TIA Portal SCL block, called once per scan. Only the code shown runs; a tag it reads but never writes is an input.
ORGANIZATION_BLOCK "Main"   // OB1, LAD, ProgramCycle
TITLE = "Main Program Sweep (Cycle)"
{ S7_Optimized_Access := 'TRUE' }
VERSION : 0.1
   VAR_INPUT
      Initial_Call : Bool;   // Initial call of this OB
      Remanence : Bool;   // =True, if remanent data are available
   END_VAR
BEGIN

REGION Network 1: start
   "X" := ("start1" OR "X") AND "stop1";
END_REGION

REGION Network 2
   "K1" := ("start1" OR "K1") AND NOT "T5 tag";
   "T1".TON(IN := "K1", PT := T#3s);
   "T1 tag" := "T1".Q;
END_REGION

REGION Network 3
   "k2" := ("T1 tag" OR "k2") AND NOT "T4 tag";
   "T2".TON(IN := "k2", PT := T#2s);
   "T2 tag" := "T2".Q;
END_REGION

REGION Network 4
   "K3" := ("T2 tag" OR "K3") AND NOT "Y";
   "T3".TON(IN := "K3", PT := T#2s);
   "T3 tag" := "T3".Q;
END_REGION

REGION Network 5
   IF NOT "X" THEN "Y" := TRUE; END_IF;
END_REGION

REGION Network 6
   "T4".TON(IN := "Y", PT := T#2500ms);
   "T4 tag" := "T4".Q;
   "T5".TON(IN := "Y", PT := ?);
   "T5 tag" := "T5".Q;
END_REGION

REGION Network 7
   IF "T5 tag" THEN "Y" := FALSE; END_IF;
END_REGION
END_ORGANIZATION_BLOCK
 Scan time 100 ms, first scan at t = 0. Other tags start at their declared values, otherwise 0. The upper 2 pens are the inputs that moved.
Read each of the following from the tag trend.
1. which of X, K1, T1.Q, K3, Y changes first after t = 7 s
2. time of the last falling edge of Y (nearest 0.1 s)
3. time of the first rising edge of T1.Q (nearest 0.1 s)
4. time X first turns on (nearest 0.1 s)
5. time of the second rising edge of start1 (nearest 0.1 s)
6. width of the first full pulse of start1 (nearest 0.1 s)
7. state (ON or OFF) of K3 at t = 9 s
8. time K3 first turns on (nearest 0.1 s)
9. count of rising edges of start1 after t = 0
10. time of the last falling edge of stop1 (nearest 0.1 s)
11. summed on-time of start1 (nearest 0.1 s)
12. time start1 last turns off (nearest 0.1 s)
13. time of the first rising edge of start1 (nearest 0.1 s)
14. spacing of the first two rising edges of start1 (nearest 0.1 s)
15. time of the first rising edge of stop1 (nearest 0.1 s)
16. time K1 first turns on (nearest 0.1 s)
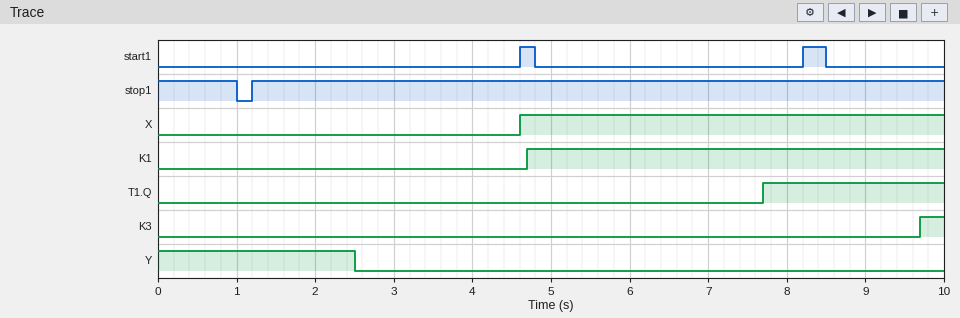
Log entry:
T1.Q
2.5 s
7.7 s
4.6 s
8.2 s
0.2 s
OFF
9.7 s
2
1.0 s
0.5 s
8.5 s
4.6 s
3.6 s
1.2 s
4.7 s
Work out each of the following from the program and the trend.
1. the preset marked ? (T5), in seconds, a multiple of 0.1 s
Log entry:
2.5 s
